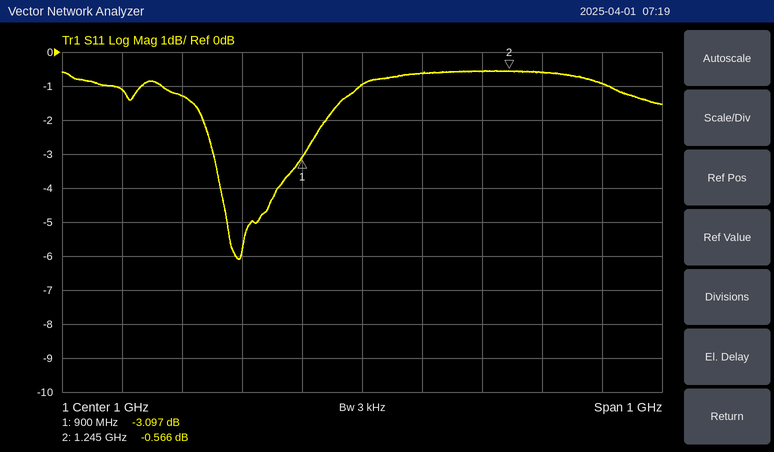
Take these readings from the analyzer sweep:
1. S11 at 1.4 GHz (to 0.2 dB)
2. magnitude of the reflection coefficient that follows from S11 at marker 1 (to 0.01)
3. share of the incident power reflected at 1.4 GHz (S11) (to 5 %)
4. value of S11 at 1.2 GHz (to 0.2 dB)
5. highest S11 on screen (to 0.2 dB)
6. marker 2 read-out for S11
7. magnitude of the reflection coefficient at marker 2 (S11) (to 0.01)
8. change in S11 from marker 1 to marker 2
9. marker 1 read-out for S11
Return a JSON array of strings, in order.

["-1.0 dB", "0.70", "80 %", "-0.6 dB", "-0.6 dB", "-0.566 dB", "0.94", "2.531 dB", "-3.097 dB"]
